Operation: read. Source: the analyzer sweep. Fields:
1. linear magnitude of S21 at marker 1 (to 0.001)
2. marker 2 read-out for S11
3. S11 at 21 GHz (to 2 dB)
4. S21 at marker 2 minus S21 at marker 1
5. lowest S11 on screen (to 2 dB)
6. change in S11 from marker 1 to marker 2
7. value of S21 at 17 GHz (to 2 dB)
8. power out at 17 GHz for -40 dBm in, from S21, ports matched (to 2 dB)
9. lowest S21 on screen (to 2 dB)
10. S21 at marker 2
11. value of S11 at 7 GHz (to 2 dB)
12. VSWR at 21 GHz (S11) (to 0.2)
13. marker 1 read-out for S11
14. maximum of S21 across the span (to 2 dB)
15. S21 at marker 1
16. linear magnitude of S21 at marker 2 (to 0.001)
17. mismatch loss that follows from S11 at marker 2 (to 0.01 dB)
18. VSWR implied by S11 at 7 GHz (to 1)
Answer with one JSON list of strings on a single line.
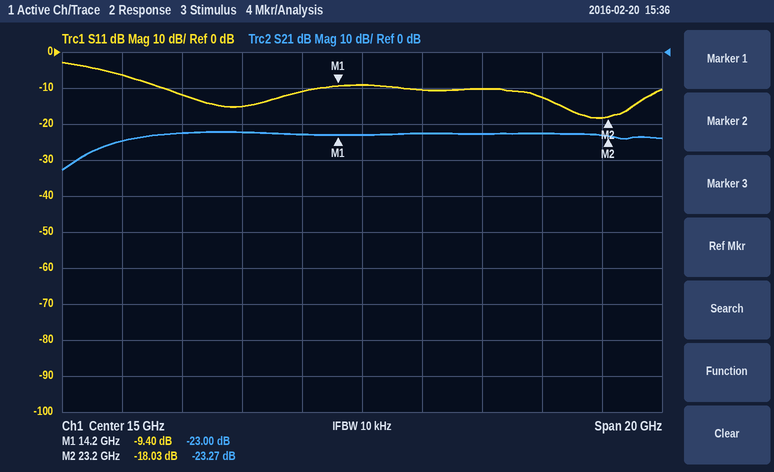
["0.071", "-18.03 dB", "-12 dB", "-0.27 dB", "-18 dB", "-8.63 dB", "-22 dB", "-62 dBm", "-32 dB", "-23.27 dB", "-6 dB", "1.6", "-9.40 dB", "-22 dB", "-23.00 dB", "0.069", "0.07 dB", "3"]
